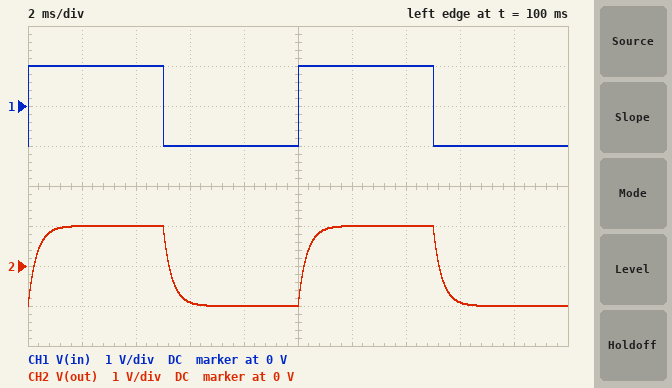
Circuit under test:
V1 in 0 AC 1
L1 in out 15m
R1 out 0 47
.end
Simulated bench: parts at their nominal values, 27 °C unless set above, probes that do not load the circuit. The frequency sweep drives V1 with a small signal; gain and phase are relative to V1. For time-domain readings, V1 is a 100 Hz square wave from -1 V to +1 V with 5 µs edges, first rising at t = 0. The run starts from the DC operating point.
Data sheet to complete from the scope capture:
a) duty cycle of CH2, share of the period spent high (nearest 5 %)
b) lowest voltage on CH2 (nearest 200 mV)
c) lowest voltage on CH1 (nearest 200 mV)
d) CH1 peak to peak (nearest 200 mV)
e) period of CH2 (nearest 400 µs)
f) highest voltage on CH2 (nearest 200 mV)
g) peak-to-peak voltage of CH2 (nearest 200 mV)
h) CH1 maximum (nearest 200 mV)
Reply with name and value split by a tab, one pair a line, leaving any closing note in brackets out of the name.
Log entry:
duty cycle of CH2, share of the period spent high	50 %
lowest voltage on CH2	-1.0 V
lowest voltage on CH1	-1.0 V
CH1 peak to peak	2.0 V
period of CH2	10.0 ms
highest voltage on CH2	1.0 V
peak-to-peak voltage of CH2	2.0 V
CH1 maximum	1.0 V
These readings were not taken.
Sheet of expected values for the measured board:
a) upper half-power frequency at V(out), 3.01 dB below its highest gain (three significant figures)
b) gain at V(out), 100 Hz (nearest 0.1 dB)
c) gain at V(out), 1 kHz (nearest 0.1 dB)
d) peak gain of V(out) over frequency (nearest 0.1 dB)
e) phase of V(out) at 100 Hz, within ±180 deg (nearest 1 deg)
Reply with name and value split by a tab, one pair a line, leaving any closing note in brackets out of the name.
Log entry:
upper half-power frequency at V(out), 3.01 dB below its highest gain	499 Hz
gain at V(out), 100 Hz	-0.2 dB
gain at V(out), 1 kHz	-7.0 dB
peak gain of V(out) over frequency	0 dB
phase of V(out) at 100 Hz, within ±180 deg	-11 deg
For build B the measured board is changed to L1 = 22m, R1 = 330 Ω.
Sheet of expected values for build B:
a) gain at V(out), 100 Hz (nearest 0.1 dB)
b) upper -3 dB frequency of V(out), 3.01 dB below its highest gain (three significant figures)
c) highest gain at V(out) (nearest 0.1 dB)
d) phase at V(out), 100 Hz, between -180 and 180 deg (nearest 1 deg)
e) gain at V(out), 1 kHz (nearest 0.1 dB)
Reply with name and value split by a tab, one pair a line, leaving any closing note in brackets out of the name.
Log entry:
gain at V(out), 100 Hz	0 dB
upper -3 dB frequency of V(out), 3.01 dB below its highest gain	2.39 kHz
highest gain at V(out)	0 dB
phase at V(out), 100 Hz, between -180 and 180 deg	-2 deg
gain at V(out), 1 kHz	-0.7 dB
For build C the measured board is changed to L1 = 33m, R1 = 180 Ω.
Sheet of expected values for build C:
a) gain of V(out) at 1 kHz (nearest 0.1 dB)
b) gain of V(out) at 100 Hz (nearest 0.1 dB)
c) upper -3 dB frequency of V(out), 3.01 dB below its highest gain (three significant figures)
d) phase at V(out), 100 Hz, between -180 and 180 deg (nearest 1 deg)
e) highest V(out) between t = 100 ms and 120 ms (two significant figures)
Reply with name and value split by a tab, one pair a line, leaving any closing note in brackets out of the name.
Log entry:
gain of V(out) at 1 kHz	-3.7 dB
gain of V(out) at 100 Hz	-0.1 dB
upper -3 dB frequency of V(out), 3.01 dB below its highest gain	868 Hz
phase at V(out), 100 Hz, between -180 and 180 deg	-7 deg
highest V(out) between t = 100 ms and 120 ms	1.0 V
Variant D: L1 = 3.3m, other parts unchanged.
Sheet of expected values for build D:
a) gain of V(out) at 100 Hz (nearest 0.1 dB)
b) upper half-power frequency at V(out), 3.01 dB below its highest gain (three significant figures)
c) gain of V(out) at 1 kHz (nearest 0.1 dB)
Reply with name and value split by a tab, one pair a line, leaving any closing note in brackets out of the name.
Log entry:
gain of V(out) at 100 Hz	0 dB
upper half-power frequency at V(out), 3.01 dB below its highest gain	2.27 kHz
gain of V(out) at 1 kHz	-0.8 dB
